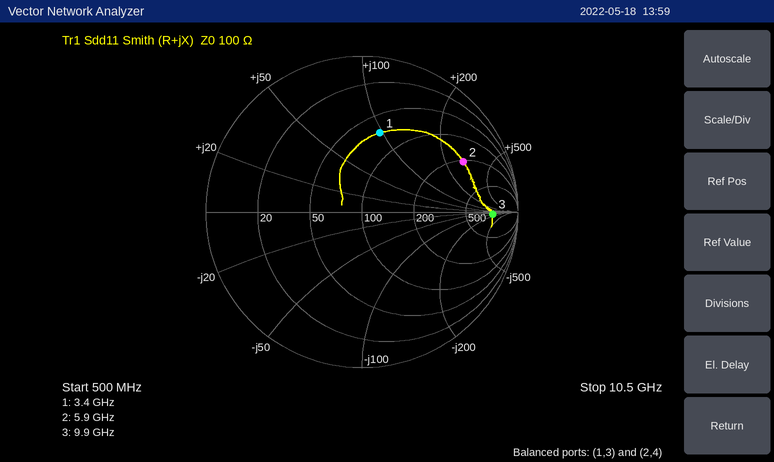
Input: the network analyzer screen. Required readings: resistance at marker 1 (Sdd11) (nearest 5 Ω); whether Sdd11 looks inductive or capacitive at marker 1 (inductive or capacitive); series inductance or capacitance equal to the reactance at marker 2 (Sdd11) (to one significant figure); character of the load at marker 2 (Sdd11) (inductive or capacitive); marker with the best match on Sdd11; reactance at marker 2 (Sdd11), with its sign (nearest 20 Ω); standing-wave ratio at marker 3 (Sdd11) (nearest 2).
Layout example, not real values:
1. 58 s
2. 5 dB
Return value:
1. 70 Ω
2. inductive
3. 8 nH
4. inductive
5. marker 1
6. +280 Ω
7. 12
